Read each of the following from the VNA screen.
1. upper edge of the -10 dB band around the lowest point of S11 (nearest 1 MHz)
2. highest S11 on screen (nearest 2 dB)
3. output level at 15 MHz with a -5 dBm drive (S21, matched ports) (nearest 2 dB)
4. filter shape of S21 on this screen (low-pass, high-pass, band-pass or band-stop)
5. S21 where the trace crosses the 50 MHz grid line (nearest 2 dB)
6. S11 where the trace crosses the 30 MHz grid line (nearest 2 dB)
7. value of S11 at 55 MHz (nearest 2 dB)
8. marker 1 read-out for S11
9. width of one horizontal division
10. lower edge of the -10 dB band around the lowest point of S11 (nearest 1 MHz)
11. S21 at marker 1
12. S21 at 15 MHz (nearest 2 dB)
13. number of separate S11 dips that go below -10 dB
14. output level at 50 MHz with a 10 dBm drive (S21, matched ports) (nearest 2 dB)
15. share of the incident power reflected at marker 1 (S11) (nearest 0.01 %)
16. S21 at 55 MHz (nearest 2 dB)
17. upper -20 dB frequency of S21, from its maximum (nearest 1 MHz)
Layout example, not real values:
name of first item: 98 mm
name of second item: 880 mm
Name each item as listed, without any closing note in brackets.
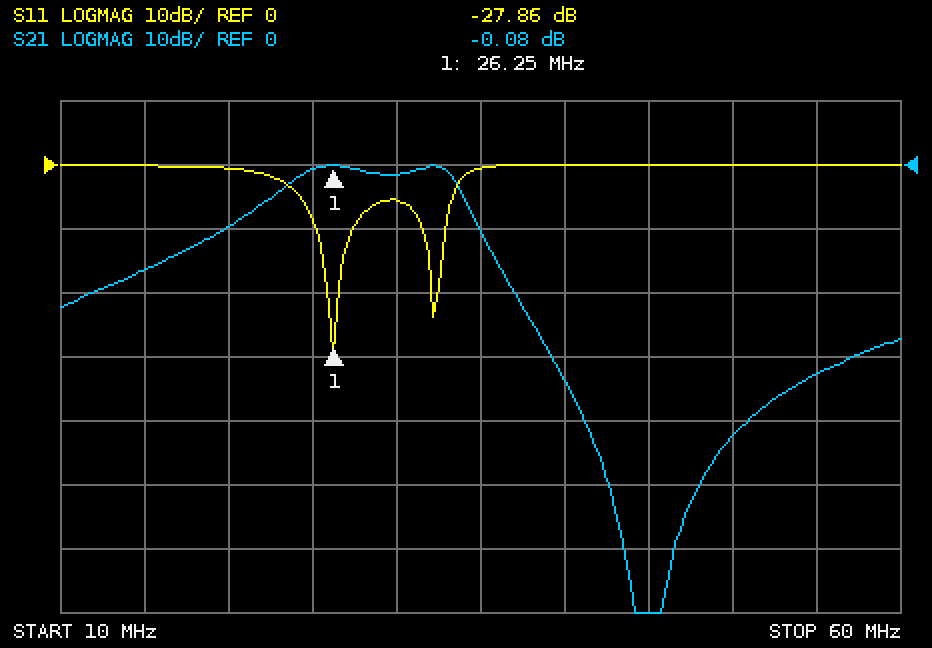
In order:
upper edge of the -10 dB band around the lowest point of S11: 27 MHz
highest S11 on screen: 0 dB
output level at 15 MHz with a -5 dBm drive (S21, matched ports): -22 dBm
filter shape of S21 on this screen: band-pass
S21 where the trace crosses the 50 MHz grid line: -42 dB
S11 where the trace crosses the 30 MHz grid line: -6 dB
value of S11 at 55 MHz: 0 dB
marker 1 read-out for S11: -27.86 dB
width of one horizontal division: 5 MHz
lower edge of the -10 dB band around the lowest point of S11: 25 MHz
S21 at marker 1: -0.08 dB
S21 at 15 MHz: -16 dB
number of separate S11 dips that go below -10 dB: 2
output level at 50 MHz with a 10 dBm drive (S21, matched ports): -32 dBm
share of the incident power reflected at marker 1 (S11): 0.16 %
S21 at 55 MHz: -32 dB
upper -20 dB frequency of S21, from its maximum: 37 MHz
